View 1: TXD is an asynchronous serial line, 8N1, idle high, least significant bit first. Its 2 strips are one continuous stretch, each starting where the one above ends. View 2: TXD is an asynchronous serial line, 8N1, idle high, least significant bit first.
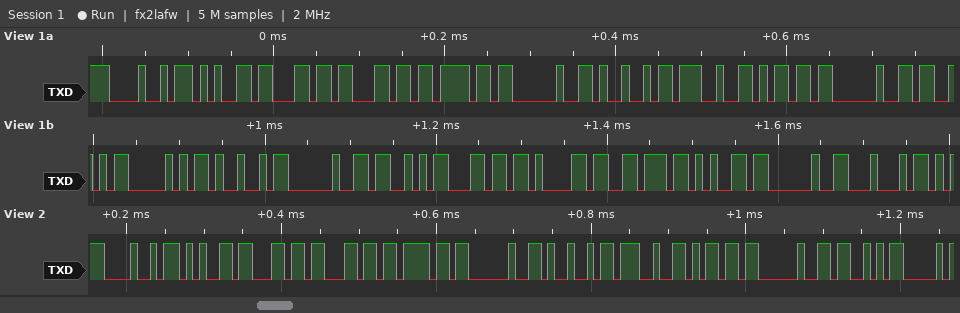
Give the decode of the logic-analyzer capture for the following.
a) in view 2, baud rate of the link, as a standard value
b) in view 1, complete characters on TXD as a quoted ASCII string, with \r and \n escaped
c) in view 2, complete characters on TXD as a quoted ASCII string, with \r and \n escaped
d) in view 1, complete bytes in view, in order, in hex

115200 baud
"Hello I'm SPI Slave D"
"Hello I'm S"
48 65 6C 6C 6F 20 49 27 6D 20 53 50 49 20 53 6C 61 76 65 20 44
